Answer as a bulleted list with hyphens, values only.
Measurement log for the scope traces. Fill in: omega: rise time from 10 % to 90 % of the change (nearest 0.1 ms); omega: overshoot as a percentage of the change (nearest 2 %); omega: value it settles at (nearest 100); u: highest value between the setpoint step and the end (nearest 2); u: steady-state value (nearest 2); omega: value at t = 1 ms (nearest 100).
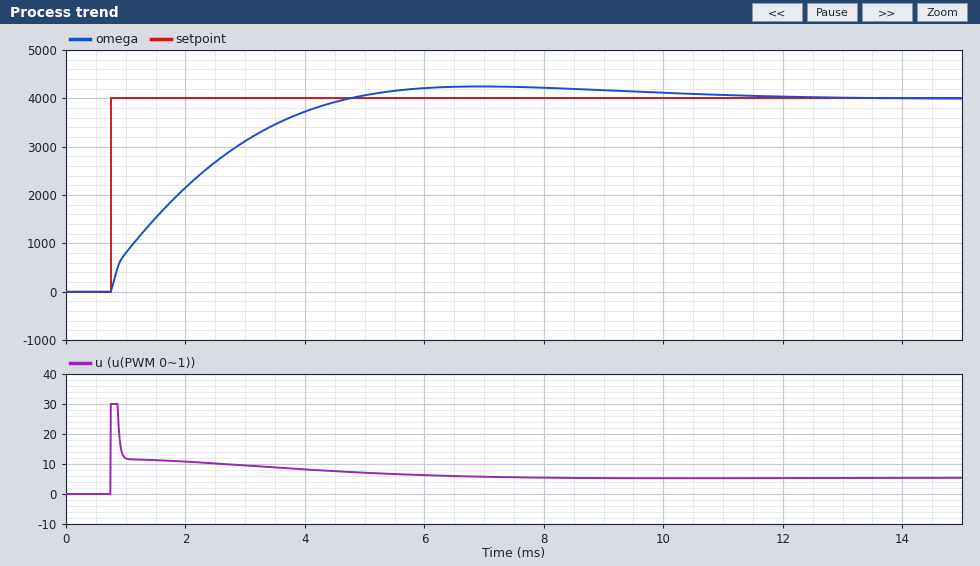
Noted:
- 2.9 ms
- 6 %
- 4000
- 30
- 6
- 800
